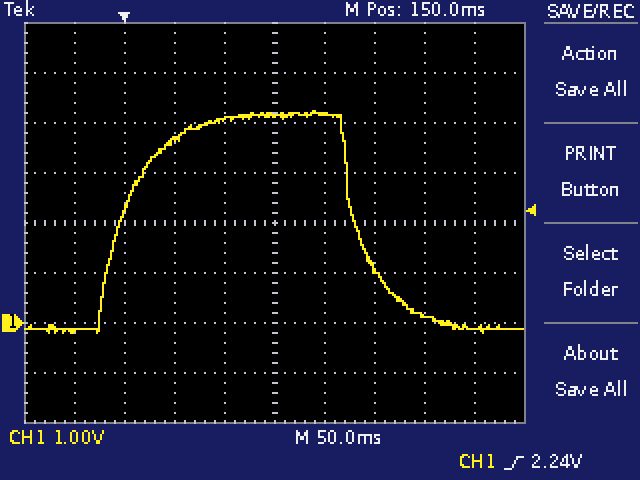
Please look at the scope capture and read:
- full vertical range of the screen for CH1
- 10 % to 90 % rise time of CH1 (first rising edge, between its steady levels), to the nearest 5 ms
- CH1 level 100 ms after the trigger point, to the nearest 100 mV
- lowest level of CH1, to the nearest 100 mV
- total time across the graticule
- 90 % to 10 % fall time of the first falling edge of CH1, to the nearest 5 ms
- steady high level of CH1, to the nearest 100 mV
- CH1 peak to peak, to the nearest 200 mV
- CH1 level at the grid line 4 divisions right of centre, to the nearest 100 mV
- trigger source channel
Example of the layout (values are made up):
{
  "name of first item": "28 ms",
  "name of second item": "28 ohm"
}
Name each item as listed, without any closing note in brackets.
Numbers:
{
  "full vertical range of the screen for CH1": "8 V",
  "10 % to 90 % rise time of CH1 (first rising edge, between its steady levels), to the nearest 5 ms": "80 ms",
  "CH1 level 100 ms after the trigger point, to the nearest 100 mV": "4.1 V",
  "lowest level of CH1, to the nearest 100 mV": "-200 mV",
  "total time across the graticule": "500 ms",
  "90 % to 10 % fall time of the first falling edge of CH1, to the nearest 5 ms": "65 ms",
  "steady high level of CH1, to the nearest 100 mV": "4.2 V",
  "CH1 peak to peak, to the nearest 200 mV": "4.4 V",
  "CH1 level at the grid line 4 divisions right of centre, to the nearest 100 mV": "-100 mV",
  "trigger source channel": "CH1"
}
